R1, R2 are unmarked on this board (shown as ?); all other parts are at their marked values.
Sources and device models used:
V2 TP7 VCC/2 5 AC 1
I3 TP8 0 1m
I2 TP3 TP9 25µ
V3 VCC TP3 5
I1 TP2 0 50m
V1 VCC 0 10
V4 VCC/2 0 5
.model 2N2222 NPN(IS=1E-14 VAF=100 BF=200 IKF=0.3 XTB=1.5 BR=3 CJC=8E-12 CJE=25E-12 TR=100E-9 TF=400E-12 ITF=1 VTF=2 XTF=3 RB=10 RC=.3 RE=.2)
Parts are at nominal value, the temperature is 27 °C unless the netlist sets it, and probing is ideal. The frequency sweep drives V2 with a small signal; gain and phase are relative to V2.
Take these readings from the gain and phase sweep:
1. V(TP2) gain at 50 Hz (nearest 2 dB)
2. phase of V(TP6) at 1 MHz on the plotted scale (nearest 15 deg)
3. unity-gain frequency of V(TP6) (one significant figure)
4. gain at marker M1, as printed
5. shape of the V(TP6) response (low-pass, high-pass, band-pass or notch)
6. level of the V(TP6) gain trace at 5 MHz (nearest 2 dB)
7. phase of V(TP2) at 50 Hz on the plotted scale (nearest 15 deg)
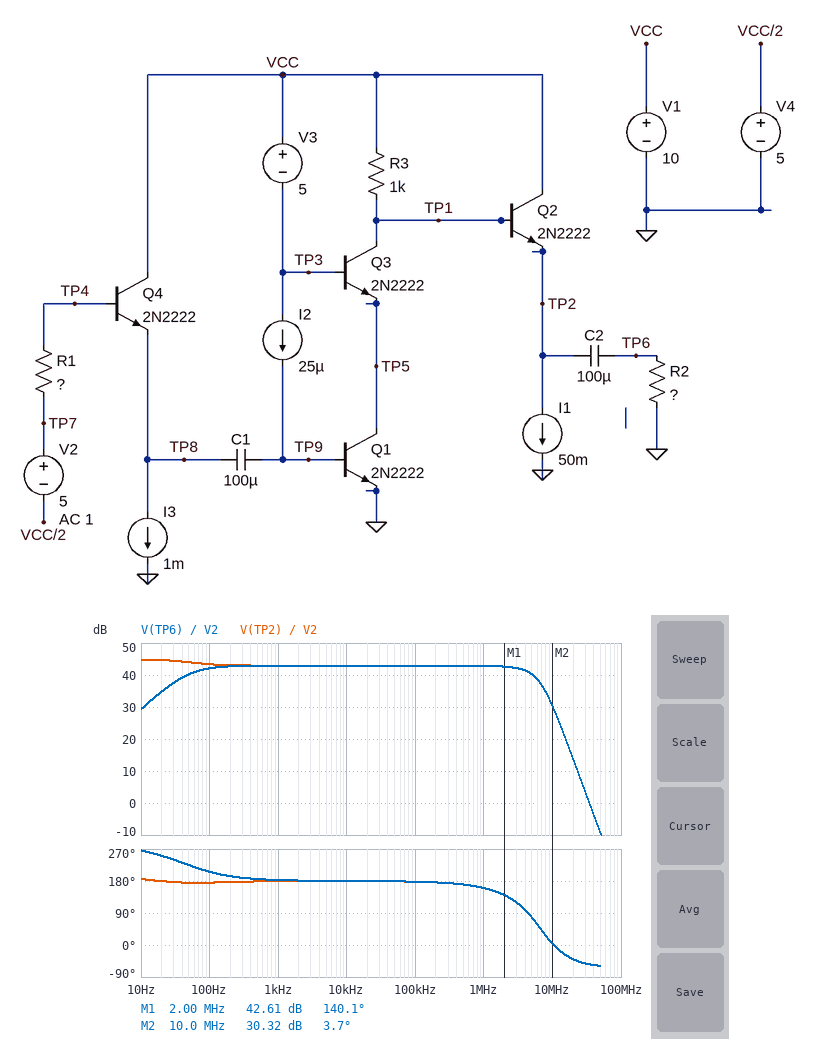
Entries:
44 dB
165 deg
30 MHz
42.61 dB
band-pass
40 dB
180 deg
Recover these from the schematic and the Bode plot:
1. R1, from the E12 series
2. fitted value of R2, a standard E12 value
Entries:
2.7 kΩ
27 Ω
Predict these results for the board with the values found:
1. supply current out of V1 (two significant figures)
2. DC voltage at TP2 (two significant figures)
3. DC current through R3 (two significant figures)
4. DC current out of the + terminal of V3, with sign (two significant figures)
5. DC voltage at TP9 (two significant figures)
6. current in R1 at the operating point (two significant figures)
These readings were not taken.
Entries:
56 mA
3.9 V
5.3 mA
-51 µA
700 mV
5.0 µA
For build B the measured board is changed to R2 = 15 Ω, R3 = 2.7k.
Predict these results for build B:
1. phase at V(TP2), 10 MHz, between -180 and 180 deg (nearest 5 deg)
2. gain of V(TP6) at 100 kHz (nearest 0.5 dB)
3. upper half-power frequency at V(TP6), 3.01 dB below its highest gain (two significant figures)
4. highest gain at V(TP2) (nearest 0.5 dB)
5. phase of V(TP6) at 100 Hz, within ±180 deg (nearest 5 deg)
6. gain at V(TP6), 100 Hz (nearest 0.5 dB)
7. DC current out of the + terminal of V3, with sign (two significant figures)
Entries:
55 deg
9.5 dB
880 kHz
10.0 dB
-135 deg
6.5 dB
-3.3 mA
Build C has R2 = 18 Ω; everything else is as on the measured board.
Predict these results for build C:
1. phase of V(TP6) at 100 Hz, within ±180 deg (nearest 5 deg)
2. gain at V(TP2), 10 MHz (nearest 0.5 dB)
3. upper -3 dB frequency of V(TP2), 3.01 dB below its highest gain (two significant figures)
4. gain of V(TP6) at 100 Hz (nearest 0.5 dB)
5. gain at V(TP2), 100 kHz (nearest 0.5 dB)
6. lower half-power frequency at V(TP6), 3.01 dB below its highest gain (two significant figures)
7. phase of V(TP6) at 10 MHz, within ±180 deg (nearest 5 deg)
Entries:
-145 deg
28.5 dB
1.6 MHz
40.5 dB
42.0 dB
64 Hz
0 deg
